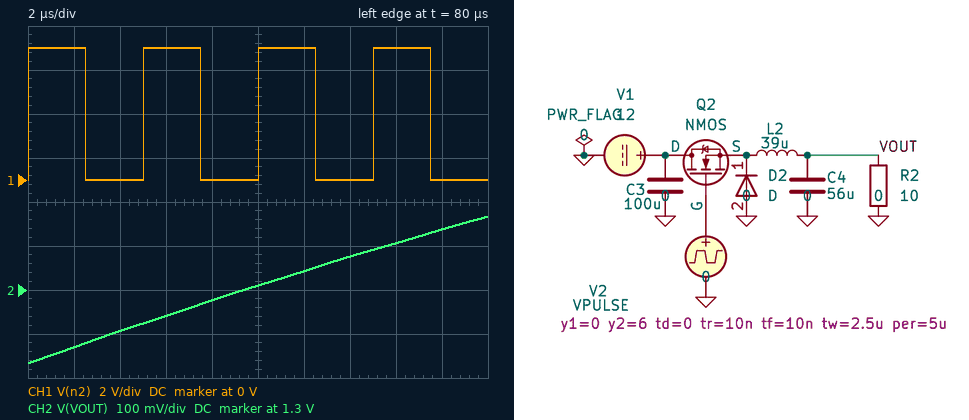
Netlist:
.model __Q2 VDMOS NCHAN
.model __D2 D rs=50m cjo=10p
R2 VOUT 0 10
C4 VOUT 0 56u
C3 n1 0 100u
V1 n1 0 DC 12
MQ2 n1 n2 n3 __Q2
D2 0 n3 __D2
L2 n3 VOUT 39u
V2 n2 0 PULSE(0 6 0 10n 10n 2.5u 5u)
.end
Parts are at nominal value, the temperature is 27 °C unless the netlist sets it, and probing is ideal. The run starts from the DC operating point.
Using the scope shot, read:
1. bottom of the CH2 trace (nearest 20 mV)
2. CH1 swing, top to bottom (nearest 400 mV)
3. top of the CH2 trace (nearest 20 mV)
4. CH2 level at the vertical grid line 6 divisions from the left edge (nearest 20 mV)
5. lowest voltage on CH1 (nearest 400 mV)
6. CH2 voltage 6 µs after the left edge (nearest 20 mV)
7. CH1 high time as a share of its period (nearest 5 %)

1.14 V
6.0 V
1.46 V
1.34 V
0 V
1.24 V
50 %
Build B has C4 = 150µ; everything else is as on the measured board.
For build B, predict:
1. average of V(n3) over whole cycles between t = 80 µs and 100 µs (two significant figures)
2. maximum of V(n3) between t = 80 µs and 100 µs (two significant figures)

880 mV
2.7 V
